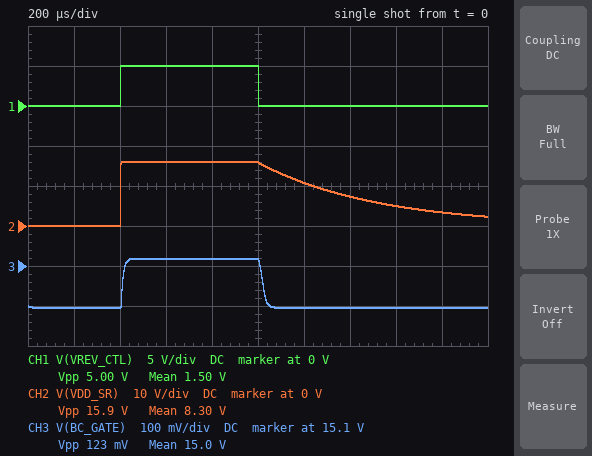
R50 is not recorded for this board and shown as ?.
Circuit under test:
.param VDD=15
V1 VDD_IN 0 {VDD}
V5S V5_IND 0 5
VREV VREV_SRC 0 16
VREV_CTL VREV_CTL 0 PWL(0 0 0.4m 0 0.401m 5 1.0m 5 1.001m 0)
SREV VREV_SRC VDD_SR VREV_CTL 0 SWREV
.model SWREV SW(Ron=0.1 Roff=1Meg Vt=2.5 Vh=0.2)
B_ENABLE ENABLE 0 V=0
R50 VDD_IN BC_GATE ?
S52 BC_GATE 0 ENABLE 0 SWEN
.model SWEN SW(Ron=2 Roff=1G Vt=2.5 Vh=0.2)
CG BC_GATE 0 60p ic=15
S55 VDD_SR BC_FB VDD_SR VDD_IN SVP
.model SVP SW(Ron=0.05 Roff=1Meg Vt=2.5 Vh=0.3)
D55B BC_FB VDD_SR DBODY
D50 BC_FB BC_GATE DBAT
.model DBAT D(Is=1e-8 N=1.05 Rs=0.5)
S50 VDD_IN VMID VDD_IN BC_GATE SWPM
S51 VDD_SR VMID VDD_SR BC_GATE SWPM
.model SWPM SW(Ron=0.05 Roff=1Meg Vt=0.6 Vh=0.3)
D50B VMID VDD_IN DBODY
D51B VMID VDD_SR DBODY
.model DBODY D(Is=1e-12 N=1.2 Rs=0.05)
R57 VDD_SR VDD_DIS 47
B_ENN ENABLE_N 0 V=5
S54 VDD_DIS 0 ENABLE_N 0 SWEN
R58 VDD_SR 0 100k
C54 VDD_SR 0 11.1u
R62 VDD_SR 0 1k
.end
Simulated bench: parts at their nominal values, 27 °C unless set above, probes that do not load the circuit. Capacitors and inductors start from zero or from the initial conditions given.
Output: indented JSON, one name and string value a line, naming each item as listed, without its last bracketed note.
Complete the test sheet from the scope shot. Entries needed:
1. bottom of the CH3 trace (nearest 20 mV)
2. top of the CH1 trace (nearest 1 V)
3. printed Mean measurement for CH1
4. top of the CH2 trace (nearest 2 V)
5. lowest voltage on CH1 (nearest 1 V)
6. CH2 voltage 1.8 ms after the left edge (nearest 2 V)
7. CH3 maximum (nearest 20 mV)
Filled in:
{
  "bottom of the CH3 trace": "15.00 V",
  "top of the CH1 trace": "5 V",
  "printed Mean measurement for CH1": "1.50 V",
  "top of the CH2 trace": "16 V",
  "lowest voltage on CH1": "0 V",
  "CH2 voltage 1.8 ms after the left edge": "4 V",
  "CH3 maximum": "15.12 V"
}
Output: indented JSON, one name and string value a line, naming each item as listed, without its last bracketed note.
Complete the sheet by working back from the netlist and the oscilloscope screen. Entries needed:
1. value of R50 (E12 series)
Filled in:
{
  "value of R50": "180 kΩ"
}
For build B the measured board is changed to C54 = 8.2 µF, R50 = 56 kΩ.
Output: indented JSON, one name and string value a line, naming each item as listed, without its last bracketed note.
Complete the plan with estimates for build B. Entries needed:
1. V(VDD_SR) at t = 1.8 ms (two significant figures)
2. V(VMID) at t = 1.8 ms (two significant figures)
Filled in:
{
  "V(VDD_SR) at t = 1.8 ms": "2.0 V",
  "V(VMID) at t = 1.8 ms": "2.5 V"
}
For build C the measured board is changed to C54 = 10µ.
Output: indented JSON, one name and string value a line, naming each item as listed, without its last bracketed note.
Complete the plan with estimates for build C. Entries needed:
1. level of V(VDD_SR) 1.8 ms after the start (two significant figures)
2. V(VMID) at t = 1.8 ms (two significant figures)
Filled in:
{
  "level of V(VDD_SR) 1.8 ms after the start": "2.9 V",
  "V(VMID) at t = 1.8 ms": "3.4 V"
}
